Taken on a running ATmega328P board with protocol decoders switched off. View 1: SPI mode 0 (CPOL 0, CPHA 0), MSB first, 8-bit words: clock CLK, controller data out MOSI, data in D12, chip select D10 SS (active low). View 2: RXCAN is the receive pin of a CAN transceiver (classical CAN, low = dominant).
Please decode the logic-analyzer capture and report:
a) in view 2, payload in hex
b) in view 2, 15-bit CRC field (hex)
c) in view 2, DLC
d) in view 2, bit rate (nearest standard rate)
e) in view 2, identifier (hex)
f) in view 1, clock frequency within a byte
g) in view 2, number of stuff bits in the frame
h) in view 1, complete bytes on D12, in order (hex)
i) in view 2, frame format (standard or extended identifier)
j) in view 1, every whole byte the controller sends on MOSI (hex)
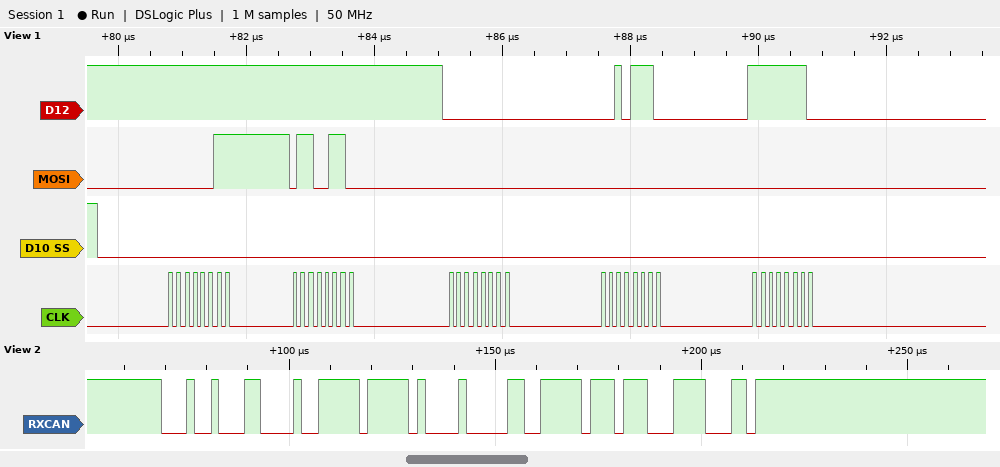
FF E1 04 FF
0x38F1
4
500 kbit/s
0x123
8 MHz
4
0xFF 0xFF 0x00 0x2E 0xFE
standard
0x03 0x66 0x00 0x00 0x00
